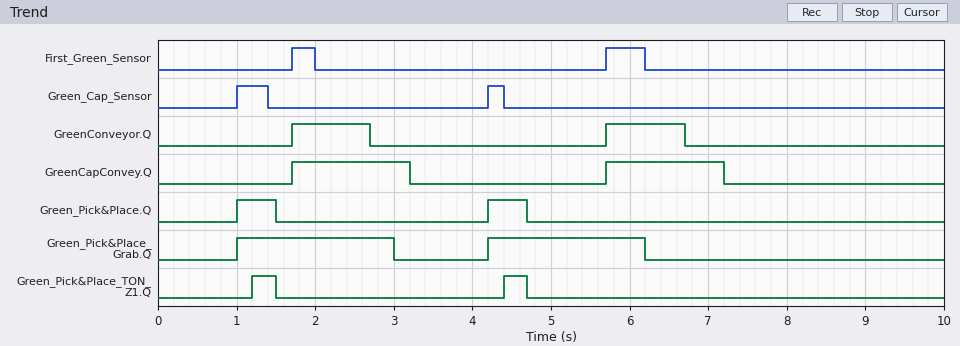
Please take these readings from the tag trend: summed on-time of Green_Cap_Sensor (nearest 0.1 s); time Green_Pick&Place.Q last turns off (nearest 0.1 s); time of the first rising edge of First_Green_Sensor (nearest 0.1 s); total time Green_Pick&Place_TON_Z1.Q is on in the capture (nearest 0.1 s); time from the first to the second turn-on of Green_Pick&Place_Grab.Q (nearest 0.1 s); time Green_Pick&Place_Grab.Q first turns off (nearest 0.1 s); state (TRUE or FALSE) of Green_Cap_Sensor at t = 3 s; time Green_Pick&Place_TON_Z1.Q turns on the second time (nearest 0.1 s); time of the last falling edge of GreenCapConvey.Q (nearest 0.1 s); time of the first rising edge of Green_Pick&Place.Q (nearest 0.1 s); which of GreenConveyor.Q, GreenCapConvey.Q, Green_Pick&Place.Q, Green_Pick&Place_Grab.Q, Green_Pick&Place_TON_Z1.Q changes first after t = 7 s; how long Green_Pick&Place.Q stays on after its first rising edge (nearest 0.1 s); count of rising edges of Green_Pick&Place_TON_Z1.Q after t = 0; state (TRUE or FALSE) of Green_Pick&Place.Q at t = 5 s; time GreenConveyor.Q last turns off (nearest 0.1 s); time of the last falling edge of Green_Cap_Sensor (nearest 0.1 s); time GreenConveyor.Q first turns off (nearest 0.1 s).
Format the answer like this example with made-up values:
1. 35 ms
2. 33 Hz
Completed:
1. 0.6 s
2. 4.7 s
3. 1.7 s
4. 0.6 s
5. 3.2 s
6. 3.0 s
7. FALSE
8. 4.4 s
9. 7.2 s
10. 1.0 s
11. GreenCapConvey.Q
12. 0.5 s
13. 2
14. FALSE
15. 6.7 s
16. 4.4 s
17. 2.7 s
